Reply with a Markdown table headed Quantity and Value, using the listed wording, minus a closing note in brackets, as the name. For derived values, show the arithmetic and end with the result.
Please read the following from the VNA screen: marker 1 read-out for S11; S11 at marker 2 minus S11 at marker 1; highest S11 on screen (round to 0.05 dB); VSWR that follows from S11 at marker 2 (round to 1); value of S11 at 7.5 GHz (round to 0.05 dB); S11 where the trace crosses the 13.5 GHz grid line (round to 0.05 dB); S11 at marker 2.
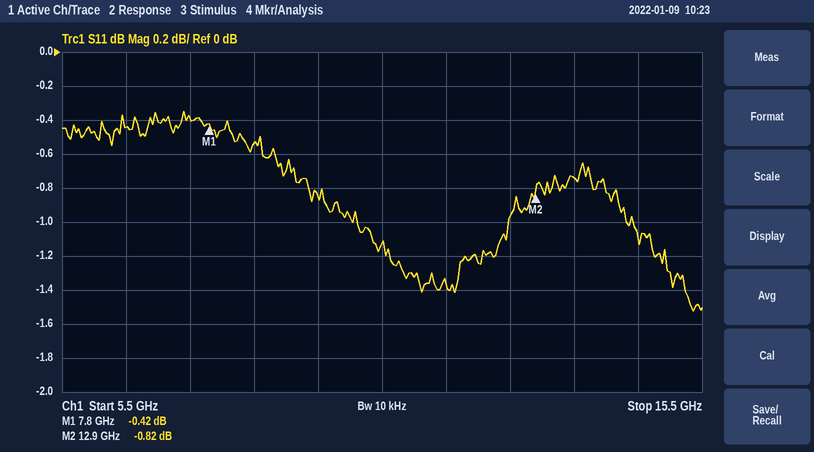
| Quantity | Value |
|---|---|
| marker 1 read-out for S11 | -0.42 dB |
| S11 at marker 2 minus S11 at marker 1 | -0.82 − (-0.42) = -0.40 dB |
| highest S11 on screen | -0.35 dB |
| VSWR that follows from S11 at marker 2 | (1 + 0.9099)/(1 − 0.9099) ≈ 21 |
| value of S11 at 7.5 GHz | -0.40 dB |
| S11 where the trace crosses the 13.5 GHz grid line | -0.75 dB |
| S11 at marker 2 | -0.82 dB |
